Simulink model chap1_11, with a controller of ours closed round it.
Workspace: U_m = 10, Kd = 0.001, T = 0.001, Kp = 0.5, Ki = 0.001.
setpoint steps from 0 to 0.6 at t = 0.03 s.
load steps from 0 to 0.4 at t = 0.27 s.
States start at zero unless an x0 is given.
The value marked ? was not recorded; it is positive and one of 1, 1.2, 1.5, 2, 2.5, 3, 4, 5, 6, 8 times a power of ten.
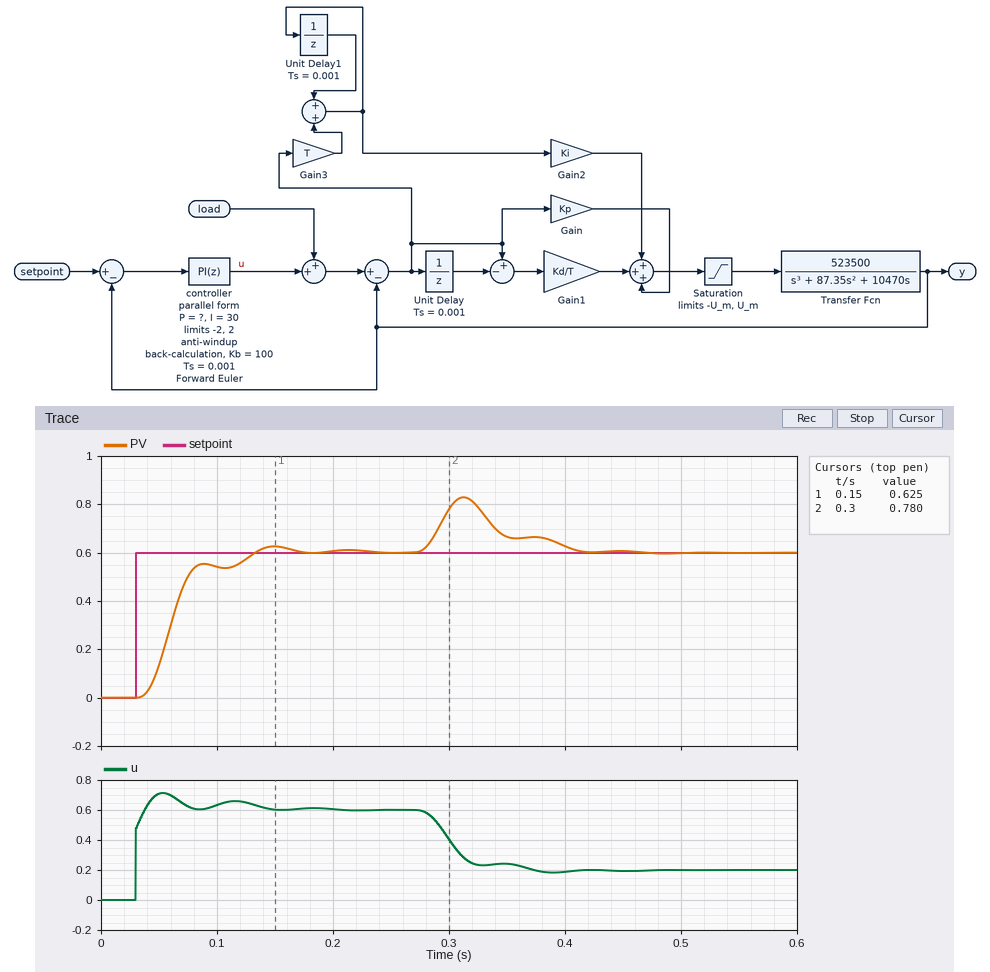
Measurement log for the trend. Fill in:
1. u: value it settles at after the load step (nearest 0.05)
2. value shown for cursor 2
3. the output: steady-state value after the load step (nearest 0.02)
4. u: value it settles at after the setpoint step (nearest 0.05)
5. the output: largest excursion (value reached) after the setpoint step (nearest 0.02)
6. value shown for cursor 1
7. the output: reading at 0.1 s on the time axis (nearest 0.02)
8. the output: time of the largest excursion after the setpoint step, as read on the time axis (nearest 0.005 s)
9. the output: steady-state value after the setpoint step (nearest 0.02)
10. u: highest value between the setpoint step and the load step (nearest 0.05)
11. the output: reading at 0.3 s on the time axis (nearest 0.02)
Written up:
0.20
0.780
0.60
0.60
0.62
0.625
0.54
0.150 s
0.60
0.70
0.78
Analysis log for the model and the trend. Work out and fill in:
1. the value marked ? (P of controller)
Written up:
0.8
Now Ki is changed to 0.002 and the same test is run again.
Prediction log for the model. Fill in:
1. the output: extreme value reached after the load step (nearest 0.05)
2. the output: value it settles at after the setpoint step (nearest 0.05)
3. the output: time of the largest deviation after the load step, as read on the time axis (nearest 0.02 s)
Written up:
0.85
0.60
0.32 s
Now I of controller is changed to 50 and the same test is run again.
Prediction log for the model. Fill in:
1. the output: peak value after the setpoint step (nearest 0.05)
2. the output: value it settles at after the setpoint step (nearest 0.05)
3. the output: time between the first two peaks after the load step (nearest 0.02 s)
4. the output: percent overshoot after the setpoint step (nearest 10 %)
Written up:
0.70
0.60
0.08 s
20 %
